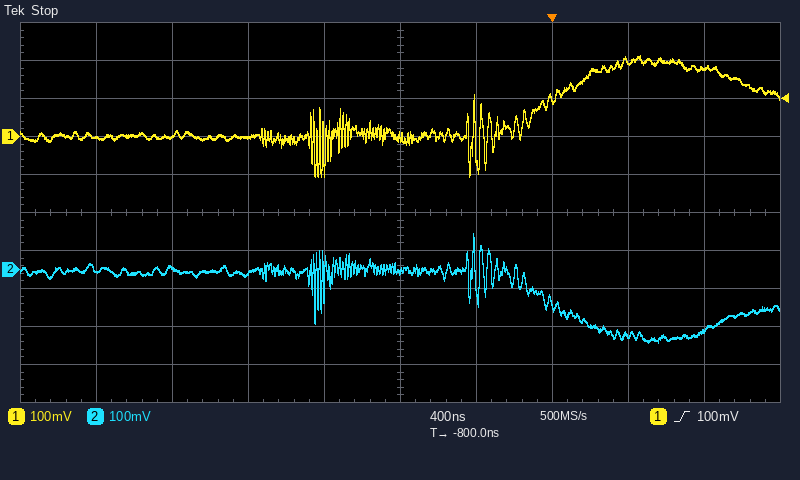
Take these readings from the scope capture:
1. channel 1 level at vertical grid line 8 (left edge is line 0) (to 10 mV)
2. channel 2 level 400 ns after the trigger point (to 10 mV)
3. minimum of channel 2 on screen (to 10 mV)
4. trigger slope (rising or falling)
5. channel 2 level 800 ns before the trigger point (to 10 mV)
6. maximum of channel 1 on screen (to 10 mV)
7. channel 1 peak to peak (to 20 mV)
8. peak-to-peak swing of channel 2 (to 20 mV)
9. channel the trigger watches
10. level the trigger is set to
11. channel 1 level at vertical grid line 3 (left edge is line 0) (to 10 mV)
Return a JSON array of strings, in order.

["200 mV", "-170 mV", "-190 mV", "rising", "0 mV", "210 mV", "320 mV", "280 mV", "channel 1", "100 mV", "0 mV"]
